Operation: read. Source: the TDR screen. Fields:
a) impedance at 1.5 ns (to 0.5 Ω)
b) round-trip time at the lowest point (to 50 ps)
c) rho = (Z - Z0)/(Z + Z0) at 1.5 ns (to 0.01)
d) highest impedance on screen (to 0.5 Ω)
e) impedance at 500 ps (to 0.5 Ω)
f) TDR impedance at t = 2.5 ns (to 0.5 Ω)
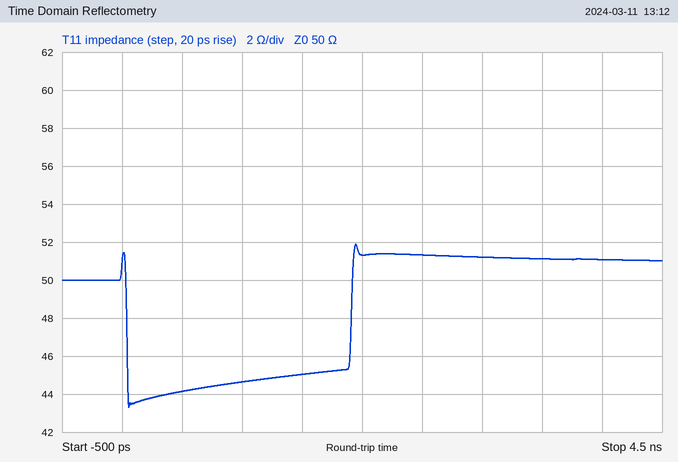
45.0 Ω
50 ps
-0.05
52.0 Ω
44.0 Ω
51.5 Ω
